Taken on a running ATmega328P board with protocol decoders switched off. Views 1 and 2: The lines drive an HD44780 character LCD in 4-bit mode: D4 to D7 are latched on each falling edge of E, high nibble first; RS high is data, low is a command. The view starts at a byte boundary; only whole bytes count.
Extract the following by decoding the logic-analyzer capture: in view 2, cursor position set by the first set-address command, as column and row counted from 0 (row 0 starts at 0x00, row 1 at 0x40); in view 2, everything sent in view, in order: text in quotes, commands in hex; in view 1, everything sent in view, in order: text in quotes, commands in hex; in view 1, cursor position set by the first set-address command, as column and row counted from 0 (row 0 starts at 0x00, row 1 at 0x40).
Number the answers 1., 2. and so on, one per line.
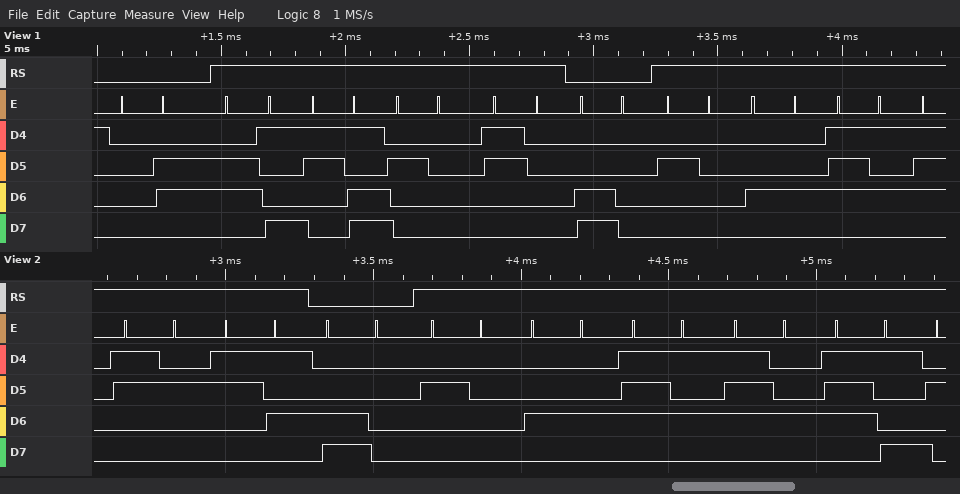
1. column 0, row 1
2. "25" 0xC0 " Duty"
3. 0x06 "i= 0" 0xC0 " Du"
4. column 0, row 1
